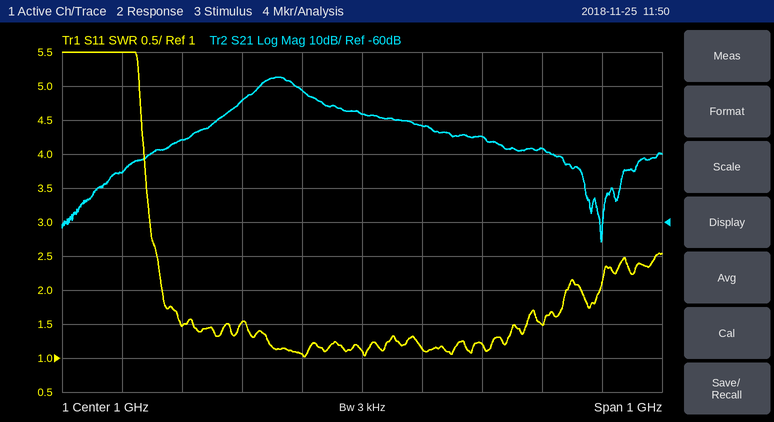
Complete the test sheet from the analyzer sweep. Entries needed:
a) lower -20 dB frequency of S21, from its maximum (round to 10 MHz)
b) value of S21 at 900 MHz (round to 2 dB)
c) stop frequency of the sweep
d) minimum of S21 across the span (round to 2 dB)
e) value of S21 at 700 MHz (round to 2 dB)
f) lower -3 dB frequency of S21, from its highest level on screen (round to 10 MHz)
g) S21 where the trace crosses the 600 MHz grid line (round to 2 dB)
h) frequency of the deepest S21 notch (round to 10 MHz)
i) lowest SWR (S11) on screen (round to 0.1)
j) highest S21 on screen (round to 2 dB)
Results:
680 MHz
-22 dB
1.5 GHz
-66 dB
-36 dB
830 MHz
-46 dB
1.40 GHz
1.0
-18 dB
